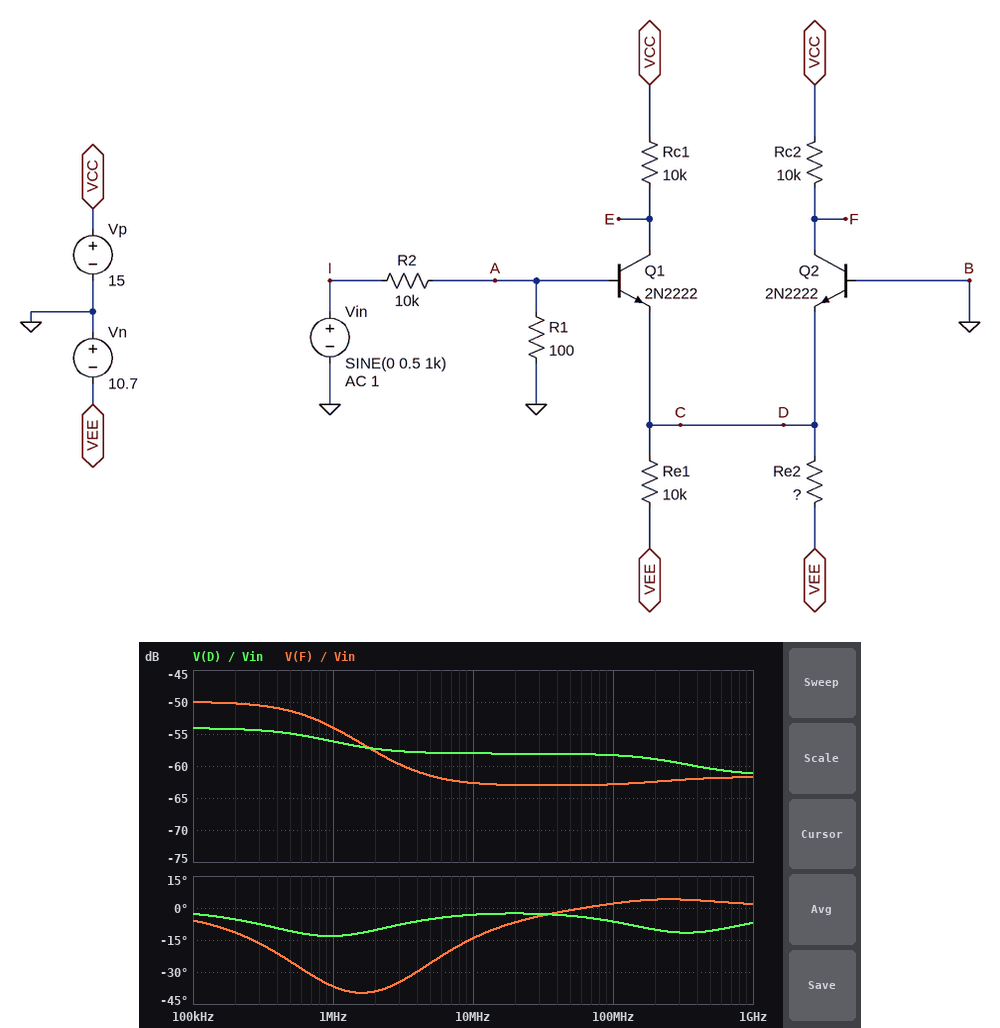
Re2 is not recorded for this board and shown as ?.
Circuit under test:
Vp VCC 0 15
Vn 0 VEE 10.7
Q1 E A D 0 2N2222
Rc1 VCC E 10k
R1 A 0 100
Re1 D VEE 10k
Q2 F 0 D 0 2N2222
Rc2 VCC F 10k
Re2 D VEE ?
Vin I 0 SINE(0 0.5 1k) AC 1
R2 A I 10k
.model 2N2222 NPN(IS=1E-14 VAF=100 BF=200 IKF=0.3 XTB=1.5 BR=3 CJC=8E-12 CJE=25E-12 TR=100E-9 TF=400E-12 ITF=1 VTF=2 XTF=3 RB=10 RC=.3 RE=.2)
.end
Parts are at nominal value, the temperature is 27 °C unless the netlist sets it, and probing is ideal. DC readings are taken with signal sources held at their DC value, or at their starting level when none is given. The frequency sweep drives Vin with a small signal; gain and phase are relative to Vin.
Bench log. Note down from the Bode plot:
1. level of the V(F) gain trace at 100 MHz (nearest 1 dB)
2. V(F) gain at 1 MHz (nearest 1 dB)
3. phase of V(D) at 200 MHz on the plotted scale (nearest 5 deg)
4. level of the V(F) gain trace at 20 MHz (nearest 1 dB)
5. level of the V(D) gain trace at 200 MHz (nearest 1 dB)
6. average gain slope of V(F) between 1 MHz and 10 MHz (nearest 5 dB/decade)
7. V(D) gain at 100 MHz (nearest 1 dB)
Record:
-63 dB
-54 dB
-10 deg
-63 dB
-59 dB
-10 dB/decade
-58 dB
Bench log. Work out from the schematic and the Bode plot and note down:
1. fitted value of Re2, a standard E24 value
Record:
3.6 kΩ
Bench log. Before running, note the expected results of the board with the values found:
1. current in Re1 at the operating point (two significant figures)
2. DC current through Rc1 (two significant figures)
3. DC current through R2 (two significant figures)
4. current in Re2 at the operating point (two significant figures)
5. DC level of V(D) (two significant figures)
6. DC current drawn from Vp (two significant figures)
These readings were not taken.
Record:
1.0 mA
1.6 mA
1.6 µA
2.8 mA
-690 mV
3.1 mA
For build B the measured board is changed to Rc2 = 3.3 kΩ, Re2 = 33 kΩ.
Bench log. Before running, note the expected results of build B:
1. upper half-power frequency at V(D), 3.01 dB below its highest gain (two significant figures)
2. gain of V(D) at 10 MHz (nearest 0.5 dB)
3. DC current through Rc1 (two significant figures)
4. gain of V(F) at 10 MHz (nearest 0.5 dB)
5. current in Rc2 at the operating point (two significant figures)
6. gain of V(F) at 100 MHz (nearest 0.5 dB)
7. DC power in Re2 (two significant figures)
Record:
2.5 MHz
-53.0 dB
640 µA
-16.5 dB
670 µA
-34.0 dB
3.1 mW
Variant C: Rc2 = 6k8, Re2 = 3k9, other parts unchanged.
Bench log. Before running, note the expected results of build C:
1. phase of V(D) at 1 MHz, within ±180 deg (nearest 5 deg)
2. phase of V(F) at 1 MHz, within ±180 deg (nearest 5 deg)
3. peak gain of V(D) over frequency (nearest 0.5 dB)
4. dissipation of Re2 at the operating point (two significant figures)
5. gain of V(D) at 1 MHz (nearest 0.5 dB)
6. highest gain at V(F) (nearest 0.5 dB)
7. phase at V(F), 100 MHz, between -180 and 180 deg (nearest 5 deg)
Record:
10 deg
-10 deg
-56.5 dB
26 mW
-59.5 dB
-7.0 dB
-110 deg
